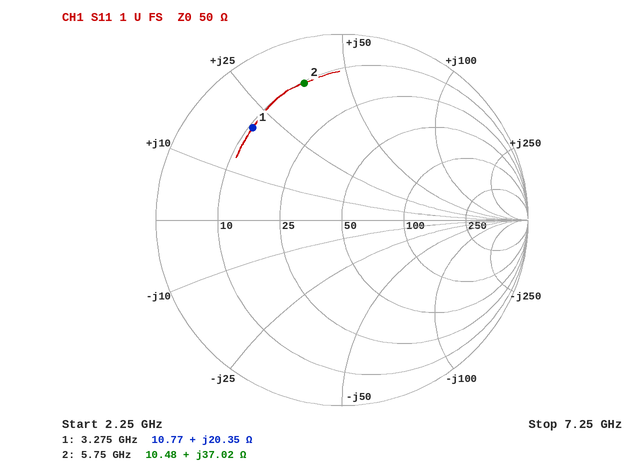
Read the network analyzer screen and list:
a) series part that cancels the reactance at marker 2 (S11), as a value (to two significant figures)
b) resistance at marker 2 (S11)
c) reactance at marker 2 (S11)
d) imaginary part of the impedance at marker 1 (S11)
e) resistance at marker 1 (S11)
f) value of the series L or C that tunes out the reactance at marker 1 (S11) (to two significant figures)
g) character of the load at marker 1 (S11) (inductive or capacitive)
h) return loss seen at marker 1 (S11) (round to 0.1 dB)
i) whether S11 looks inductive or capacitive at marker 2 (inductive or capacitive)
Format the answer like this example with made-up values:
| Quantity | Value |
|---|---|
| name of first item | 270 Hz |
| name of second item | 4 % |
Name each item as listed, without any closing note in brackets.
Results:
| Quantity | Value |
|---|---|
| series part that cancels the reactance at marker 2 (S11), as a value | 750 fF |
| resistance at marker 2 | 10.48 Ω |
| reactance at marker 2 | +37.02 Ω |
| imaginary part of the impedance at marker 1 | +20.35 Ω |
| resistance at marker 1 | 10.77 Ω |
| value of the series L or C that tunes out the reactance at marker 1 (S11) | 2.4 pF |
| character of the load at marker 1 (S11) | inductive |
| return loss seen at marker 1 (S11) | 3.2 dB |
| whether S11 looks inductive or capacitive at marker 2 | inductive |
